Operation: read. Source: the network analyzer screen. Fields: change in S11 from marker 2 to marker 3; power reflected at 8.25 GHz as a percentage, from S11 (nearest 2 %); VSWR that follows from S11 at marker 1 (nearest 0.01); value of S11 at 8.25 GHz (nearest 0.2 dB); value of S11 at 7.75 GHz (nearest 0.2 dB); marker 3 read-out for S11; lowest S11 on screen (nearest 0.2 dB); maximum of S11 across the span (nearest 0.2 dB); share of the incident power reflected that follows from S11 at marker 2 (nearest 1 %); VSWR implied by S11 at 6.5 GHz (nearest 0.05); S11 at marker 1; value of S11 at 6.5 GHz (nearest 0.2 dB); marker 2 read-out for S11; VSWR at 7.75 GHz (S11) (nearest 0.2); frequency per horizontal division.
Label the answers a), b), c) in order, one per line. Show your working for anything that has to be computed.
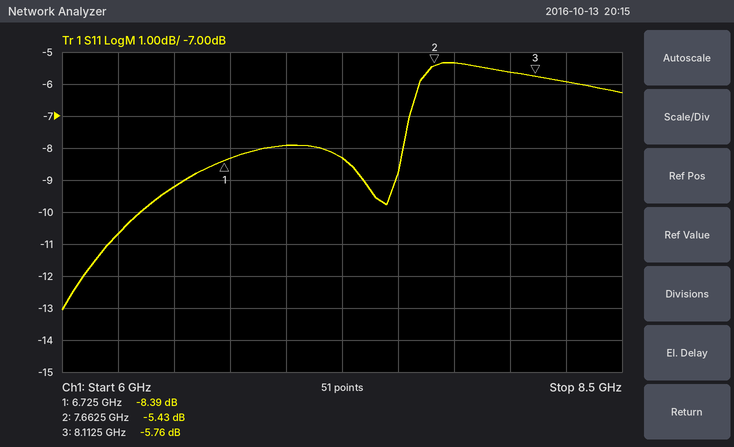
a) -5.76 − (-5.43) = -0.33 dB
b) 10^(-6/10) ≈ 25.1 %, so 26 % to the nearest 2 %
c) (1 + 0.3806)/(1 − 0.3806) ≈ 2.23
d) -6.0 dB
e) -5.4 dB
f) -5.76 dB
g) -13.0 dB
h) -5.4 dB
i) 10^(-5.43/10) ≈ 29 %
j) |Γ| = 10^(-9.2/20) = 0.3467; VSWR = (1 + 0.3467)/(1 − 0.3467) ≈ 2.06, so 2.05 to the nearest 0.05
k) -8.39 dB
l) -9.2 dB
m) -5.43 dB
n) |Γ| = 10^(-5.4/20) = 0.5370; VSWR = (1 + 0.5370)/(1 − 0.5370) ≈ 3.32, so 3.4 to the nearest 0.2
o) 250 MHz
